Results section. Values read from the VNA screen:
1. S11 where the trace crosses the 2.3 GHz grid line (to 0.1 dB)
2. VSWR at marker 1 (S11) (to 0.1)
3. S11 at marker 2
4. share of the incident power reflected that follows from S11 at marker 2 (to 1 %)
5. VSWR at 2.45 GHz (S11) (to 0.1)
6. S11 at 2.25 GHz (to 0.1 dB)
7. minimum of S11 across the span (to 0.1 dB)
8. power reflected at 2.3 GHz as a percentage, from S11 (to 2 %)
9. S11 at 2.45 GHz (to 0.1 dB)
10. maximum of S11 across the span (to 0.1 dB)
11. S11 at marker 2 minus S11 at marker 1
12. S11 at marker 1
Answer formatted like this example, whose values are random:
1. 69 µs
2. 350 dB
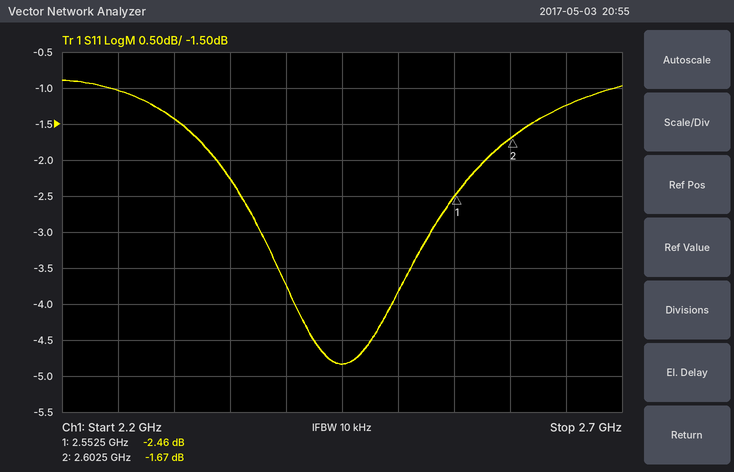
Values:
1. -1.4 dB
2. 7.1
3. -1.67 dB
4. 68 %
5. 3.7
6. -1.0 dB
7. -4.8 dB
8. 72 %
9. -4.8 dB
10. -0.9 dB
11. 0.79 dB
12. -2.46 dB
